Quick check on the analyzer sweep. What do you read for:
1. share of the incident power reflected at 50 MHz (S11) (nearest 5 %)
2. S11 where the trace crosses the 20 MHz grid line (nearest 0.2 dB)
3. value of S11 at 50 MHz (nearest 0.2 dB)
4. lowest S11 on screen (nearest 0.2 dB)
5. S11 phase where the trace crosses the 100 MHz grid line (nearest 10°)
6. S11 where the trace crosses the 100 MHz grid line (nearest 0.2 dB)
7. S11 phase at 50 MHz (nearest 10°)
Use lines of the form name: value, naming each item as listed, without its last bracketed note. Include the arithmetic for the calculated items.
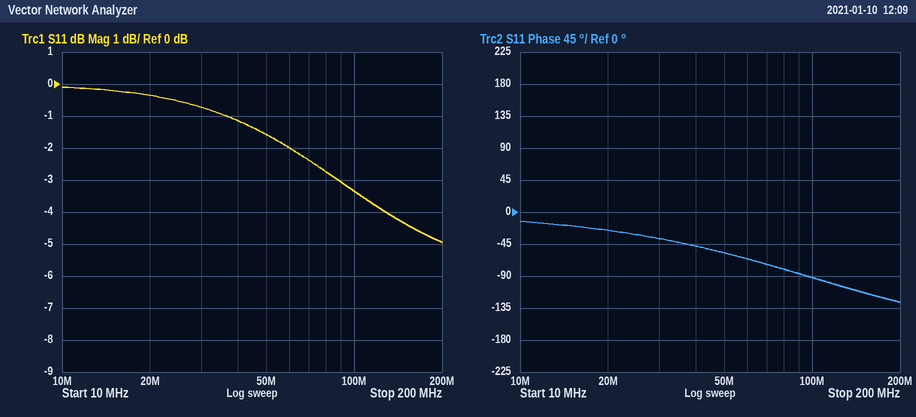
share of the incident power reflected at 50 MHz (S11): 10^(-1.6/10) ≈ 69.2 %, so 70 % to the nearest 5 %
S11 where the trace crosses the 20 MHz grid line: -0.4 dB
value of S11 at 50 MHz: -1.6 dB
lowest S11 on screen: -5.0 dB
S11 phase where the trace crosses the 100 MHz grid line: -90°
S11 where the trace crosses the 100 MHz grid line: -3.4 dB
S11 phase at 50 MHz: -60°
